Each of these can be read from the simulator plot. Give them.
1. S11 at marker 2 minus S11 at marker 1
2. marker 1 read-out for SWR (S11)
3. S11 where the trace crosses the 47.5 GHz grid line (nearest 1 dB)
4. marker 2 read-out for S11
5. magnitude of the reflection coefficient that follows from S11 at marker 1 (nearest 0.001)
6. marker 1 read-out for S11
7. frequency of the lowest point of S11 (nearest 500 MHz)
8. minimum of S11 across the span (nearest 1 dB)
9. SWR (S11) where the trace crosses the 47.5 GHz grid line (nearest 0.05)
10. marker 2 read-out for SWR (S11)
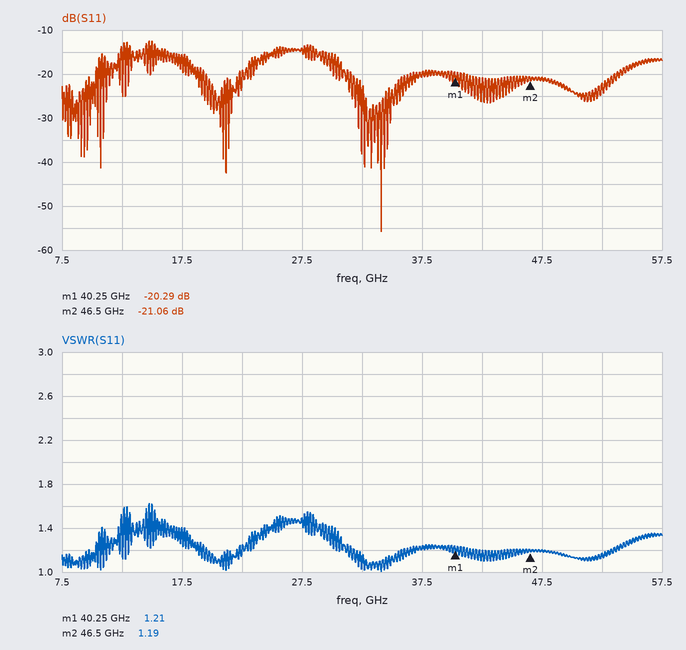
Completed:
-0.77 dB
1.21
-21 dB
-21.06 dB
0.097
-20.29 dB
34.0 GHz
-56 dB
1.20
1.19
